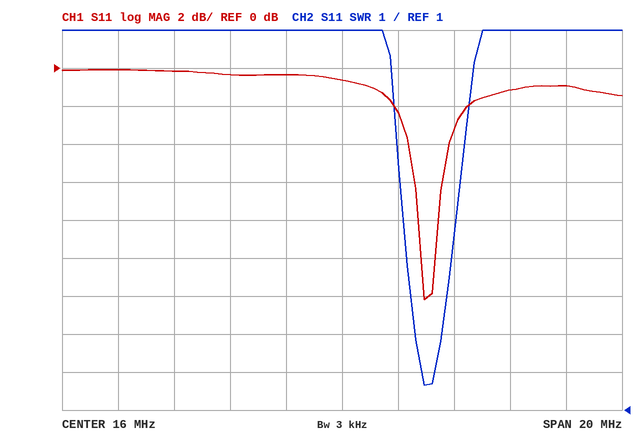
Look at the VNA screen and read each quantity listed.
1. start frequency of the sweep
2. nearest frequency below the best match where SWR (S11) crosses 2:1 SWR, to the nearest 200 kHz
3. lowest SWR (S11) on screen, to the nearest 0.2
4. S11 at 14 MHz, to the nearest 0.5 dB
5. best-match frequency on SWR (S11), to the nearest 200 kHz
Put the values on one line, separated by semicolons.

6 MHz; 18.8 MHz; 1.6; -0.5 dB; 19.0 MHz
